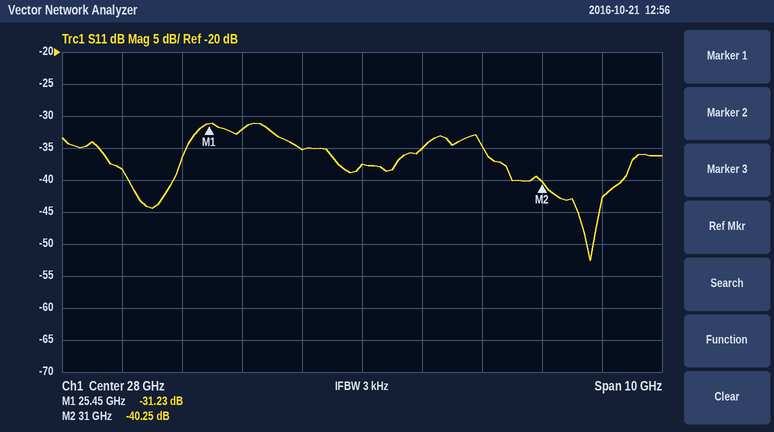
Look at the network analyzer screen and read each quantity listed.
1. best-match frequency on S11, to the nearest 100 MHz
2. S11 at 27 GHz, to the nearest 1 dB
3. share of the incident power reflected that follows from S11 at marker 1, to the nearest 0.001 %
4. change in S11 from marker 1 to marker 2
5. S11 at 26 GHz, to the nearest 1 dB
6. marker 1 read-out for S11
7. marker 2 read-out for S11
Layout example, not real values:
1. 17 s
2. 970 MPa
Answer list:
1. 31.8 GHz
2. -35 dB
3. 0.075 %
4. -9.02 dB
5. -32 dB
6. -31.23 dB
7. -40.25 dB
